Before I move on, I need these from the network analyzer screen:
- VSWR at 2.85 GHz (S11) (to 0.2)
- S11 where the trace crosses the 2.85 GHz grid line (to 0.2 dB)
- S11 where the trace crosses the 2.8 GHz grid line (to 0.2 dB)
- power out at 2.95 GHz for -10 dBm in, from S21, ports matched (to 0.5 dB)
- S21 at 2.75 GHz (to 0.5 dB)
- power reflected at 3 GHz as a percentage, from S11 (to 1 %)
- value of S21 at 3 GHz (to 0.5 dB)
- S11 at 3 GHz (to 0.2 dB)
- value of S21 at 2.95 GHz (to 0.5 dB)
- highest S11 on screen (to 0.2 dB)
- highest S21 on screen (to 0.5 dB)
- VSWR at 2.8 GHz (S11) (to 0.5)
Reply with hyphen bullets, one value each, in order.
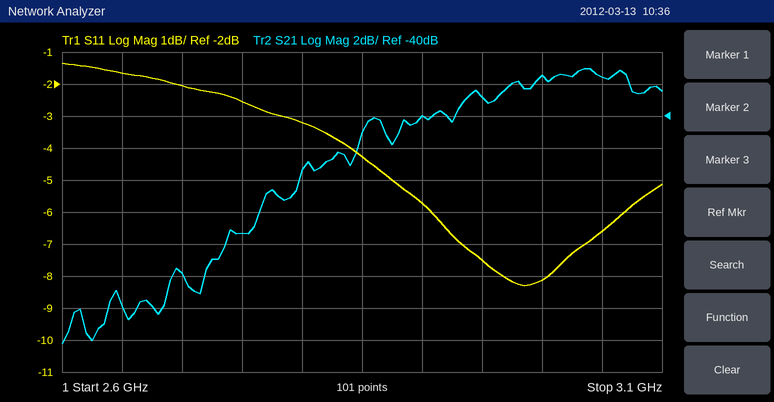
- 4.2
- -4.2 dB
- -3.2 dB
- -49.0 dBm
- -47.5 dB
- 15 %
- -37.5 dB
- -8.2 dB
- -39.0 dB
- -1.4 dB
- -37.0 dB
- 5.5
